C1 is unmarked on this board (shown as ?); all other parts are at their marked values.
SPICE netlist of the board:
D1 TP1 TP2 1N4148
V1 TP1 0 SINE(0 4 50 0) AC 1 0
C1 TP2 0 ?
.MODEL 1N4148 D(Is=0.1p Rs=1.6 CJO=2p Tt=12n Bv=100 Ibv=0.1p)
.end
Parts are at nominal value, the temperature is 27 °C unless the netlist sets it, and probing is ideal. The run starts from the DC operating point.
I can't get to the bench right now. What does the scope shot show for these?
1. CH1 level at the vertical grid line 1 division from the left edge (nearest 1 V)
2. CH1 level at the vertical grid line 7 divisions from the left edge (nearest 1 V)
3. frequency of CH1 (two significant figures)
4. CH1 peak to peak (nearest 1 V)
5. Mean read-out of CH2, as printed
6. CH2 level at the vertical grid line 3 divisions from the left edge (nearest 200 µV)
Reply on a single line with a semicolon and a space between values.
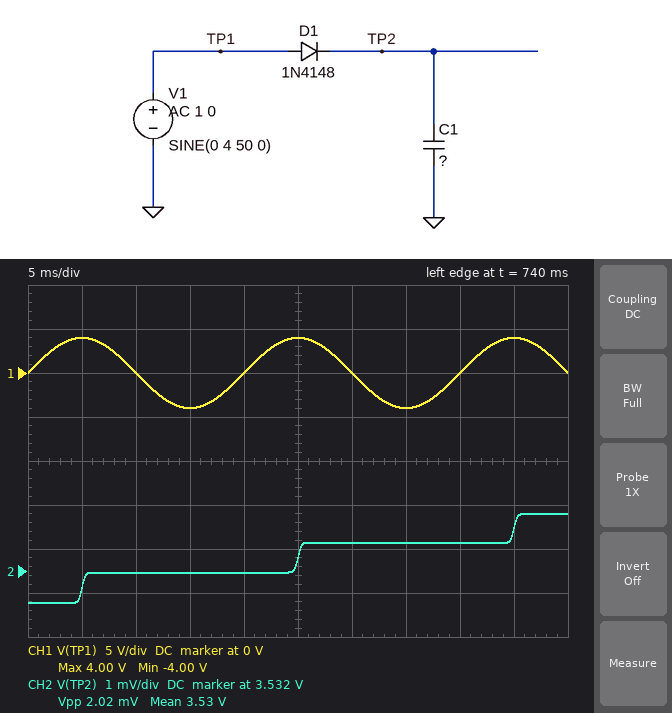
4 V; -4 V; 50 Hz; 8 V; 3.53 V; 3.5320 V
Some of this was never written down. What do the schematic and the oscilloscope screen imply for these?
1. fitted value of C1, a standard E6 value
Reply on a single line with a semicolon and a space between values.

6.8 µF
